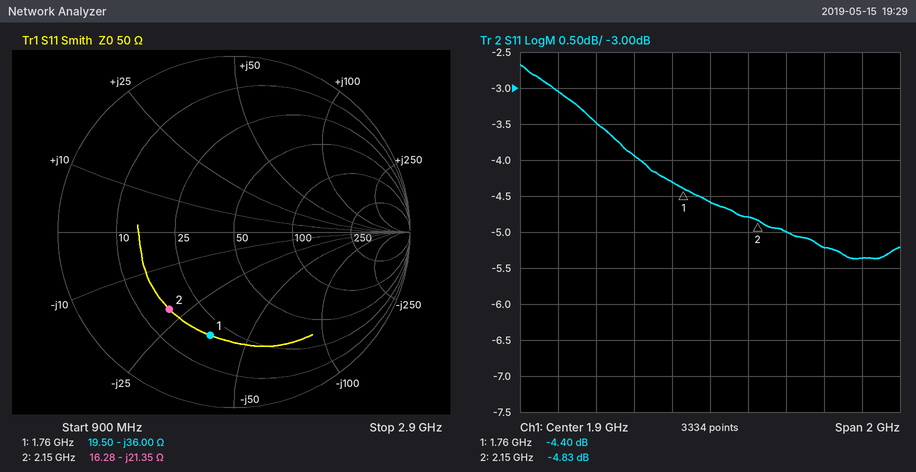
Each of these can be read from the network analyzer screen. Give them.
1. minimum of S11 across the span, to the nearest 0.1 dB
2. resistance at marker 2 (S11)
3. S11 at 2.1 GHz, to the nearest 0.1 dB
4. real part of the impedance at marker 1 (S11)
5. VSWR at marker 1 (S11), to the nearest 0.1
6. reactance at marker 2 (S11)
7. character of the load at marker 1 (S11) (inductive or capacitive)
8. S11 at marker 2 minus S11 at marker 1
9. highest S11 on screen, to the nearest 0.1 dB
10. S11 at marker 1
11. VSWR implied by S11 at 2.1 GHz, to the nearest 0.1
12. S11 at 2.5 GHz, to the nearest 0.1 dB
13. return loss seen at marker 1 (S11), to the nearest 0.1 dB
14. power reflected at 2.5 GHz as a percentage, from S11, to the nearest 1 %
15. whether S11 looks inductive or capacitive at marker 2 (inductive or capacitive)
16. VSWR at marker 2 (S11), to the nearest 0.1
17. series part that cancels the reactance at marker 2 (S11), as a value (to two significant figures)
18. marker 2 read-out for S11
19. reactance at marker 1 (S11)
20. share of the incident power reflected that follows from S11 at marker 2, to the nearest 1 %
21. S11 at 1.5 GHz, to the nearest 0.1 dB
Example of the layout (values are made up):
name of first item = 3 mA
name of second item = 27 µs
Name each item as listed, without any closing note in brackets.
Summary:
minimum of S11 across the span, to the nearest 0.1 dB = -5.4 dB
resistance at marker 2 = 16.28 Ω
S11 at 2.1 GHz, to the nearest 0.1 dB = -4.8 dB
real part of the impedance at marker 1 = 19.50 Ω
VSWR at marker 1 (S11), to the nearest 0.1 = 4.0
reactance at marker 2 = -21.35 Ω
character of the load at marker 1 (S11) = capacitive
S11 at marker 2 minus S11 at marker 1 = -0.43 dB
highest S11 on screen, to the nearest 0.1 dB = -2.7 dB
S11 at marker 1 = -4.40 dB
VSWR implied by S11 at 2.1 GHz, to the nearest 0.1 = 3.7
S11 at 2.5 GHz, to the nearest 0.1 dB = -5.2 dB
return loss seen at marker 1 (S11), to the nearest 0.1 dB = 4.4 dB
power reflected at 2.5 GHz as a percentage, from S11, to the nearest 1 % = 30 %
whether S11 looks inductive or capacitive at marker 2 = capacitive
VSWR at marker 2 (S11), to the nearest 0.1 = 3.7
series part that cancels the reactance at marker 2 (S11), as a value = 1.6 nH
marker 2 read-out for S11 = -4.83 dB
reactance at marker 1 = -36.00 Ω
share of the incident power reflected that follows from S11 at marker 2, to the nearest 1 % = 33 %
S11 at 1.5 GHz, to the nearest 0.1 dB = -3.9 dB
